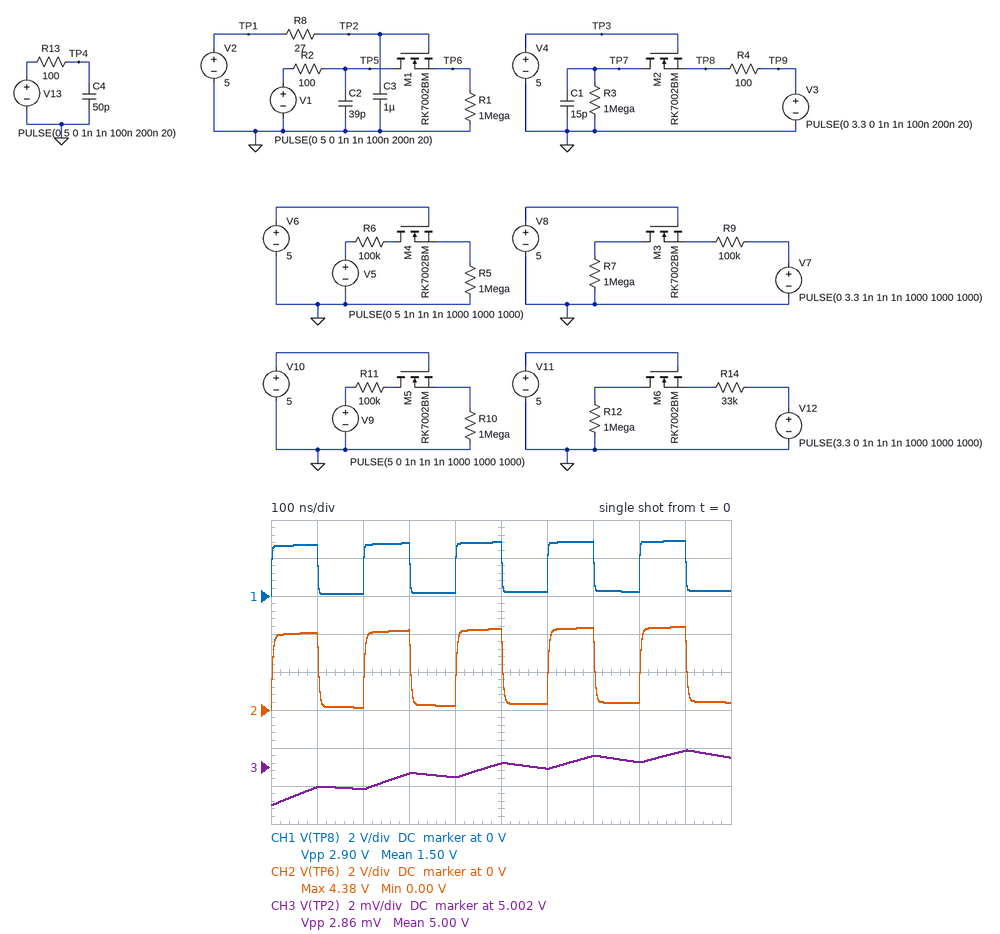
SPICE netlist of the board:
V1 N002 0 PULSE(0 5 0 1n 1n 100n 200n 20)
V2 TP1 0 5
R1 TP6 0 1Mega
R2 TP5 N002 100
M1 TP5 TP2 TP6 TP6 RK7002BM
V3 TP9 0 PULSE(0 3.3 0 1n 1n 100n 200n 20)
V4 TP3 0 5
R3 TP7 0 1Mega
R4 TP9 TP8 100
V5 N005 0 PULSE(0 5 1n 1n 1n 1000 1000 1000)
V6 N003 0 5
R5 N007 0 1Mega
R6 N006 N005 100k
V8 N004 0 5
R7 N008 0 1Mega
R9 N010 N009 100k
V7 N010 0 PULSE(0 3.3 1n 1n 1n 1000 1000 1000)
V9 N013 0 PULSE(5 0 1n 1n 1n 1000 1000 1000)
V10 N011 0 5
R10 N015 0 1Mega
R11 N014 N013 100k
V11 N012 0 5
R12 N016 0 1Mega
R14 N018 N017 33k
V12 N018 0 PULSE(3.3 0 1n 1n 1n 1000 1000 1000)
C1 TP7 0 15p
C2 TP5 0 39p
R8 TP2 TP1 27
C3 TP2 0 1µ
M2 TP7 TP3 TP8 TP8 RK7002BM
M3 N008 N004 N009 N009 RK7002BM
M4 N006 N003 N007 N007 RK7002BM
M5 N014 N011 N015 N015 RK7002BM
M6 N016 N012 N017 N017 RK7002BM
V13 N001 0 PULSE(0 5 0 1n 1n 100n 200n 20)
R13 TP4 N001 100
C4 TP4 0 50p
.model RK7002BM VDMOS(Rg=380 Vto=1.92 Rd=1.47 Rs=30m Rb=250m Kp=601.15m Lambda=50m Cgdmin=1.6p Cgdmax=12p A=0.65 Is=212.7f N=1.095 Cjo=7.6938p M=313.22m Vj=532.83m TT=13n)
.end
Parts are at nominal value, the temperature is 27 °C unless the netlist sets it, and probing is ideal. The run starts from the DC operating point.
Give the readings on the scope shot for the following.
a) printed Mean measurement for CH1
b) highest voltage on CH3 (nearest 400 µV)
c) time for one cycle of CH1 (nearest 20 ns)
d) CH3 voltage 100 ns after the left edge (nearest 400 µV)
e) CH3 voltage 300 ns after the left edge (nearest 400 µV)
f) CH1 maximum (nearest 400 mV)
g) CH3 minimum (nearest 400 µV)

1.50 V
5.0028 V
200 ns
5.0008 V
5.0016 V
2.8 V
5.0000 V
